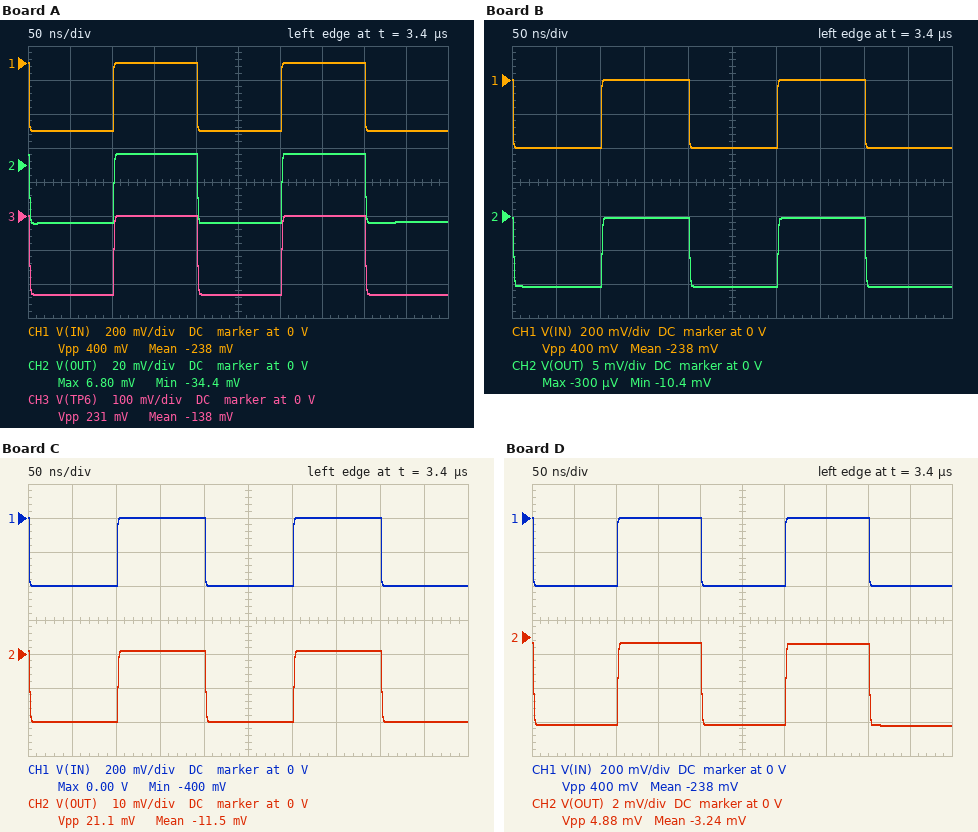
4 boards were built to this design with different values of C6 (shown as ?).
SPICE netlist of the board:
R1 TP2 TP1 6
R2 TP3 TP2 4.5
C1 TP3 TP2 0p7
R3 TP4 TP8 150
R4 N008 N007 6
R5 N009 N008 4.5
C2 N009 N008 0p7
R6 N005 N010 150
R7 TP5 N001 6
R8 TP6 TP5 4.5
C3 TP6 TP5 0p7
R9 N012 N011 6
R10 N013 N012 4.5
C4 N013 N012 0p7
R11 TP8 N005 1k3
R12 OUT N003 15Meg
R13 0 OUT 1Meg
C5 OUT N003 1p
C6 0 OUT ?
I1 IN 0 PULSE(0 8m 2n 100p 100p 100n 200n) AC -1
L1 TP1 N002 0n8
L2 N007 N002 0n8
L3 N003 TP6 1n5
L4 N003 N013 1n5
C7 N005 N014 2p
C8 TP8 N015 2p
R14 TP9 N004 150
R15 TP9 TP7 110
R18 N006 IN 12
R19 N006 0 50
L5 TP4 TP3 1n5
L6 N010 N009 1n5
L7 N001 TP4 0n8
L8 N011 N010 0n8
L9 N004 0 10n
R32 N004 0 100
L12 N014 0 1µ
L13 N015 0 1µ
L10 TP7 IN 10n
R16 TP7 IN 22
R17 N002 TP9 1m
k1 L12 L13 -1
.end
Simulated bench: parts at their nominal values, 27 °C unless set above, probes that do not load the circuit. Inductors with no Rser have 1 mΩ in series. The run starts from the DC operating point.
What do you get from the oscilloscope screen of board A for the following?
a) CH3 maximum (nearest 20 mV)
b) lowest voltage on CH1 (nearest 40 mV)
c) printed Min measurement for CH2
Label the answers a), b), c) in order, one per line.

a) 0 V
b) -400 mV
c) -34.4 mV
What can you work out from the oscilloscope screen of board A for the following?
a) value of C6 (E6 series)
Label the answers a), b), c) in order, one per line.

a) 4.7 pF
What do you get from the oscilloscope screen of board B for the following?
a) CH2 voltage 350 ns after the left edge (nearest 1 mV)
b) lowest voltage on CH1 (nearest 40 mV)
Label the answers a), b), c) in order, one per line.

a) 0 V
b) -400 mV
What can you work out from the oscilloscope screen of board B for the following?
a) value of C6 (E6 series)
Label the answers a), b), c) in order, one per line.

a) 22 pF
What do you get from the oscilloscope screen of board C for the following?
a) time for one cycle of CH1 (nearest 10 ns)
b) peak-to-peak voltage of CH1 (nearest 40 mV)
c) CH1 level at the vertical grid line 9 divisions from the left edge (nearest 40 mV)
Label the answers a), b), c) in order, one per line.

a) 200 ns
b) 400 mV
c) -400 mV
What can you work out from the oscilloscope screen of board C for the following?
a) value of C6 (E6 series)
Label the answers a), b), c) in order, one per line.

a) 10 pF
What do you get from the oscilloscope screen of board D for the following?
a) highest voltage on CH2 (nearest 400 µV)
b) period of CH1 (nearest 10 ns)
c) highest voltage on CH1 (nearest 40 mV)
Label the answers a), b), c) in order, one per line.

a) -400 µV
b) 200 ns
c) 0 V
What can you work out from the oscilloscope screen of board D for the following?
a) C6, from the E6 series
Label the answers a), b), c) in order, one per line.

a) 47 pF
